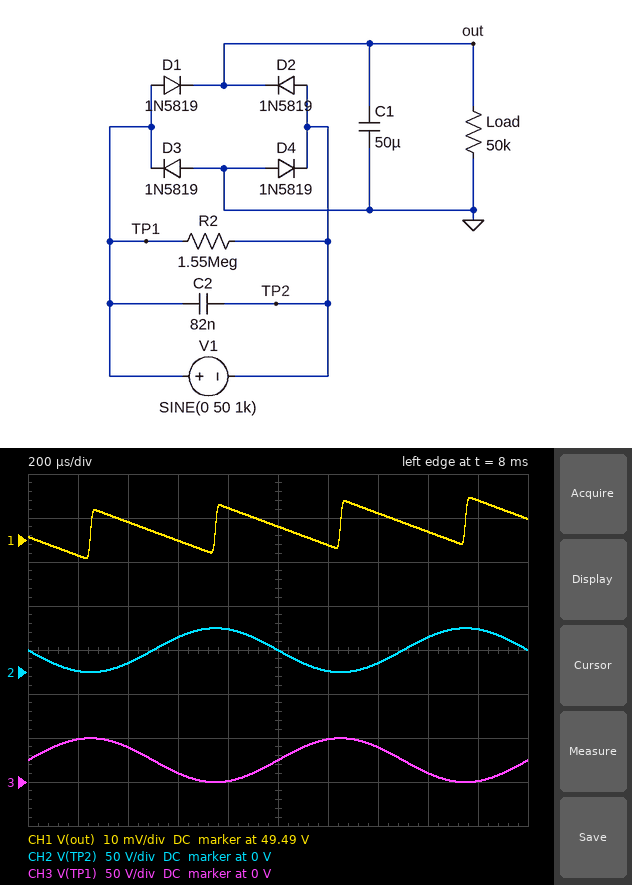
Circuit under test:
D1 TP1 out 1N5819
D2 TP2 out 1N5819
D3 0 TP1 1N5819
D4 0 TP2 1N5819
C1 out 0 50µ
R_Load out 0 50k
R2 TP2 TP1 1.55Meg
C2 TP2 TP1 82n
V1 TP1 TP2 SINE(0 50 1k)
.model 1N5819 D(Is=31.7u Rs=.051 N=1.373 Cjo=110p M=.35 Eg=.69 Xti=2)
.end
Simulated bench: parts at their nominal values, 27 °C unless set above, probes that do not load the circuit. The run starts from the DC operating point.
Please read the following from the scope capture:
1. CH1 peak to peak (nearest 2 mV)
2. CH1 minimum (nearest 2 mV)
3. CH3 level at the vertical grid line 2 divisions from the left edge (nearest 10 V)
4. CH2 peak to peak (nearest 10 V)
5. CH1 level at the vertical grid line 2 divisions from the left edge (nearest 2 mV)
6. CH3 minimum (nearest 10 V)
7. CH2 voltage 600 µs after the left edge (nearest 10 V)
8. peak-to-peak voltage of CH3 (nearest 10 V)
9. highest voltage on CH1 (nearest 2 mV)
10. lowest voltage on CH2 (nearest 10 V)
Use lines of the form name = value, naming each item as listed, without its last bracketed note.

CH1 peak to peak = 14 mV
CH1 minimum = 49.486 V
CH3 level at the vertical grid line 2 divisions from the left edge = 40 V
CH2 peak to peak = 50 V
CH1 level at the vertical grid line 2 divisions from the left edge = 49.494 V
CH3 minimum = 0 V
CH2 voltage 600 µs after the left edge = 40 V
peak-to-peak voltage of CH3 = 50 V
highest voltage on CH1 = 49.500 V
lowest voltage on CH2 = 0 V
